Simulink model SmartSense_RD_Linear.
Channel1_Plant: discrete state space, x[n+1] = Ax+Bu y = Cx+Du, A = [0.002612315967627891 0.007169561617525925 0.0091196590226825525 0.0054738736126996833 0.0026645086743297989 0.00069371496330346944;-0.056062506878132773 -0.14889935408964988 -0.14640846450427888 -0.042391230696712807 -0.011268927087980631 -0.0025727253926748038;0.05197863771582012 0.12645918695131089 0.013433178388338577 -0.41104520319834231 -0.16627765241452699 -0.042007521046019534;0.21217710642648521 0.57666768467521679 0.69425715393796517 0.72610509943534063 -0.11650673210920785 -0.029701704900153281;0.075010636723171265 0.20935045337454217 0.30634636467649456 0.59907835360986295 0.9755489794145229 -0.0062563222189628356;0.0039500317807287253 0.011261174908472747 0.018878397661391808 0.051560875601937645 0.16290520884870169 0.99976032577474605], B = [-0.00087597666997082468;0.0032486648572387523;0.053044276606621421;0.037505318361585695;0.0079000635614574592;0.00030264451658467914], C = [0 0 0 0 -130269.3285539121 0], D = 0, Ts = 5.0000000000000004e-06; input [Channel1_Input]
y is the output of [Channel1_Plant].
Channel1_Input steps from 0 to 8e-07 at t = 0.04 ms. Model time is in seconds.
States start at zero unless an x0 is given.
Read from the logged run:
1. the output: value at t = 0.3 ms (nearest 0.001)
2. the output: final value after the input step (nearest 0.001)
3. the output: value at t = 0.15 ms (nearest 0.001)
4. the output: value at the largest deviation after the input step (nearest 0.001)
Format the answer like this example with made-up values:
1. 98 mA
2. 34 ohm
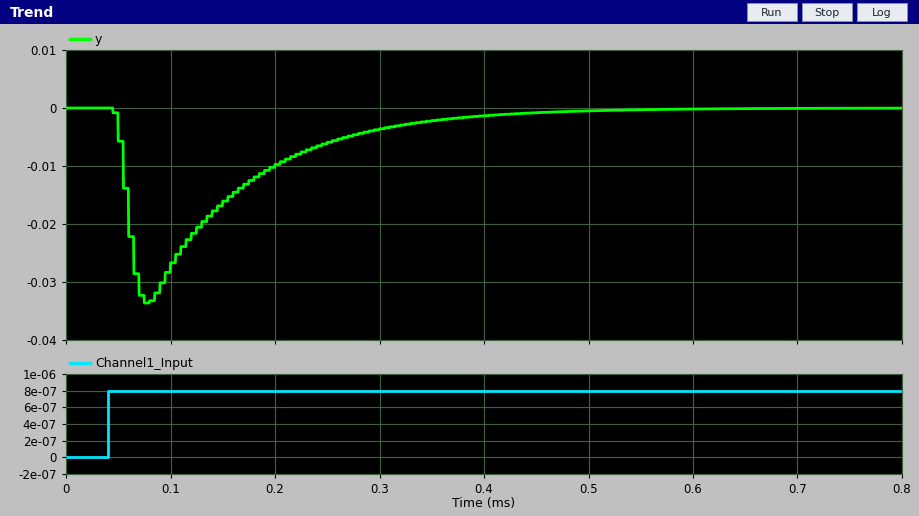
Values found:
1. -0.004
2. 0.000
3. -0.016
4. -0.034
